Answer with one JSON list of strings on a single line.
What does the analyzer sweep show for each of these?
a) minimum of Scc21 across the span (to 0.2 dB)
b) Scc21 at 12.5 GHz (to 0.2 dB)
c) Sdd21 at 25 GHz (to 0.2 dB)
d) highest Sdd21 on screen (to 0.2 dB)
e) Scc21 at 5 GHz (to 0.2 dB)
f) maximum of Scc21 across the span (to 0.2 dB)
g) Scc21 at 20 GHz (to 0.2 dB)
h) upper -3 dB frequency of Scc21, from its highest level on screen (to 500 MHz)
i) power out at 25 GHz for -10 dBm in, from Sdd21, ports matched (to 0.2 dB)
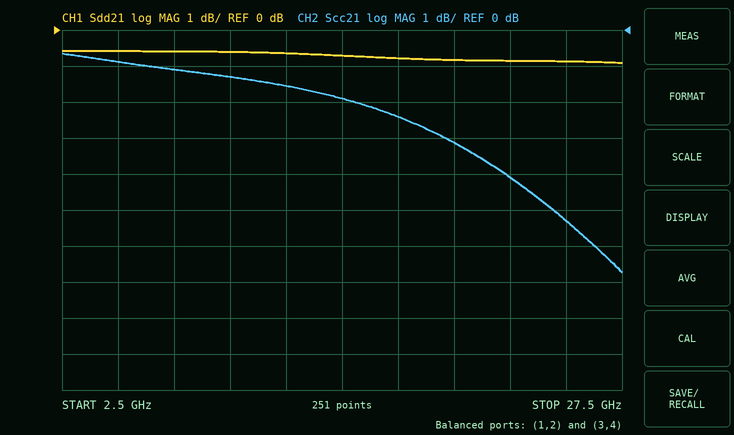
["-6.8 dB", "-1.6 dB", "-0.8 dB", "-0.6 dB", "-0.8 dB", "-0.6 dB", "-3.2 dB", "21.5 GHz", "-10.8 dBm"]
